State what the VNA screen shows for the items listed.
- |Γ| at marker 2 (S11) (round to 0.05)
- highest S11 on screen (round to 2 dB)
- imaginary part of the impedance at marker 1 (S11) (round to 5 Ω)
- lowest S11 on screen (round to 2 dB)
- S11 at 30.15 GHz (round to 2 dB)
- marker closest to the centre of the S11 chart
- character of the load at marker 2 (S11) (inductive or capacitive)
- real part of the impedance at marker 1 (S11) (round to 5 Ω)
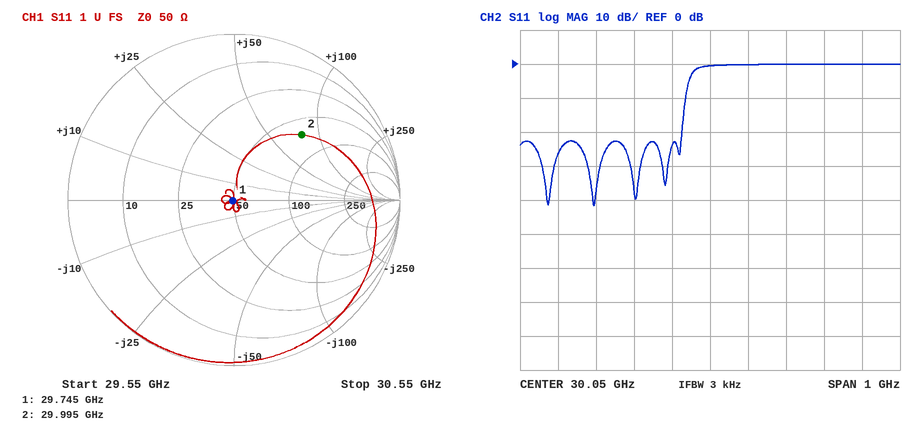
0.55
0 dB
0 Ω
-42 dB
0 dB
marker 1
inductive
50 Ω
